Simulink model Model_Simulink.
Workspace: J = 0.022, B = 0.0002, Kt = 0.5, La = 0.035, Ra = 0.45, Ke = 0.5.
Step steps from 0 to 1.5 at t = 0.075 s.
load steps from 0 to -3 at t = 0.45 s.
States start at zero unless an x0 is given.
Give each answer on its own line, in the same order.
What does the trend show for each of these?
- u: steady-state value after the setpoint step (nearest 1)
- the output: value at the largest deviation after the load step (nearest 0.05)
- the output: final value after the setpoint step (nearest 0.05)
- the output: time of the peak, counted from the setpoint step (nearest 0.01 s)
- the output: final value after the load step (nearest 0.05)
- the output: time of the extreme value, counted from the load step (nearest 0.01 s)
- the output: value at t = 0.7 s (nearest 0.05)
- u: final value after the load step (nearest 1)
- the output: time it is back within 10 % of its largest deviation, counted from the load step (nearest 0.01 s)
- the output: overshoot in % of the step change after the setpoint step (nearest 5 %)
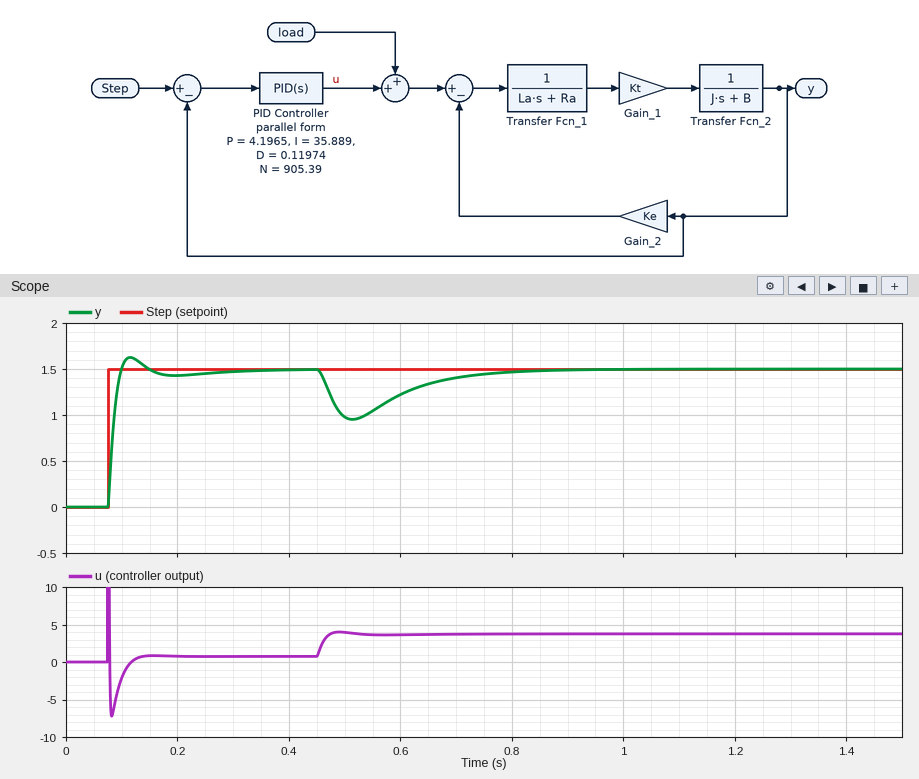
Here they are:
1
0.95
1.50
0.04 s
1.50
0.06 s
1.40
4
0.30 s
10 %
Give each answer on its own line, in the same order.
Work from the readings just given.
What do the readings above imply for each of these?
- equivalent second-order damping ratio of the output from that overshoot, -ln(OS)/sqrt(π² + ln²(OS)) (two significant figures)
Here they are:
0.59
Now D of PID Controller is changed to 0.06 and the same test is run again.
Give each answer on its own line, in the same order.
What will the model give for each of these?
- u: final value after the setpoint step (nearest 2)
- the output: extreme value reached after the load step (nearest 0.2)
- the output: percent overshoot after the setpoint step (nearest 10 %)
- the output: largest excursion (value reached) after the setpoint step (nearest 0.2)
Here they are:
0
0.8
20 %
1.8
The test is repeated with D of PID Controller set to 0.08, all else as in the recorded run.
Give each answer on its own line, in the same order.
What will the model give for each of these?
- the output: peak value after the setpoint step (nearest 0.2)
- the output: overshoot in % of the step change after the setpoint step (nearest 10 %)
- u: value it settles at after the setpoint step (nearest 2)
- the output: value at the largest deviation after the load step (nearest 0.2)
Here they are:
1.8
20 %
0
0.8
